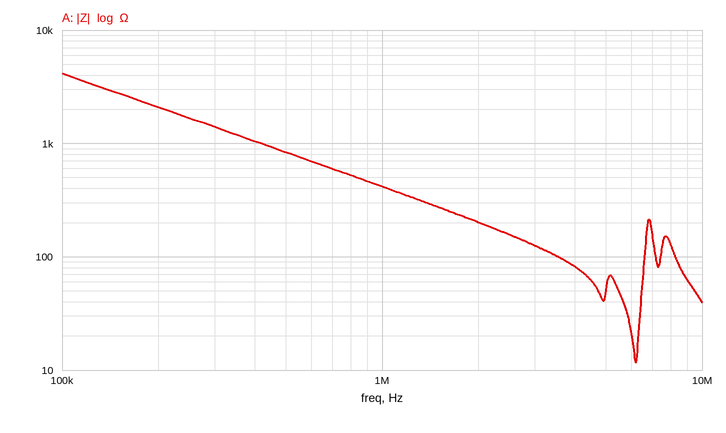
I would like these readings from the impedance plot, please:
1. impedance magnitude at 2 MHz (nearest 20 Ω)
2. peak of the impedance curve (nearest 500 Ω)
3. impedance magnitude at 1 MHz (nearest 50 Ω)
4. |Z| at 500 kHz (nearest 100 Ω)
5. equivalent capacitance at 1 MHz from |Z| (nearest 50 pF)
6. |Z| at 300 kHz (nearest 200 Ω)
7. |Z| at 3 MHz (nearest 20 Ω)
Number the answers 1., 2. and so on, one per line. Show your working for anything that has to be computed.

1. 200 Ω
2. 4.0 kΩ
3. 400 Ω
4. 800 Ω
5. C = 1/(2π × 1 MHz × 400 Ω) ≈ 398 pF, so 400 pF to the nearest 50 pF
6. 1.4 kΩ
7. 120 Ω
